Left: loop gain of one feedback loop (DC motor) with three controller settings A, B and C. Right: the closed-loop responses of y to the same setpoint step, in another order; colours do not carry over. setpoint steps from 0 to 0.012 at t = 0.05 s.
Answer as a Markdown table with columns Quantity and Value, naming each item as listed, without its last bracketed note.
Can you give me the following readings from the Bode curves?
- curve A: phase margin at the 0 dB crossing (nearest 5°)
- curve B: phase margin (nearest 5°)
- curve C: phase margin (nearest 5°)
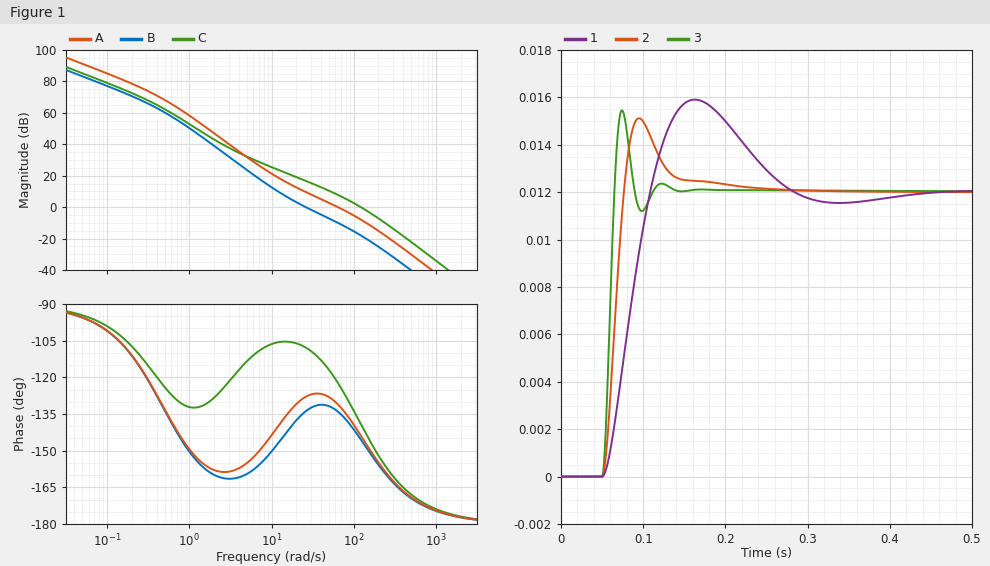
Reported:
| Quantity | Value |
|---|---|
| curve A: phase margin at the 0 dB crossing | 50° |
| curve B: phase margin | 45° |
| curve C: phase margin | 40° |
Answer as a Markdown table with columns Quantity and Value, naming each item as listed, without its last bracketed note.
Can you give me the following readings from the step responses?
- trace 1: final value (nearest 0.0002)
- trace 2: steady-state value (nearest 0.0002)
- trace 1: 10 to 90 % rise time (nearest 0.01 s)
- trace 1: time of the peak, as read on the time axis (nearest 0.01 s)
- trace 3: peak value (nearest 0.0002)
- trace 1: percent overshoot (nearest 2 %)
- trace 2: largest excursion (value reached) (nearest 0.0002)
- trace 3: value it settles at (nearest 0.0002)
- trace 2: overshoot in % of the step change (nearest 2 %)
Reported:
| Quantity | Value |
|---|---|
| trace 1: final value | 0.0120 |
| trace 2: steady-state value | 0.0120 |
| trace 1: 10 to 90 % rise time | 0.04 s |
| trace 1: time of the peak, as read on the time axis | 0.16 s |
| trace 3: peak value | 0.0154 |
| trace 1: percent overshoot | 32 % |
| trace 2: largest excursion (value reached) | 0.0152 |
| trace 3: value it settles at | 0.0120 |
| trace 2: overshoot in % of the step change | 26 % |
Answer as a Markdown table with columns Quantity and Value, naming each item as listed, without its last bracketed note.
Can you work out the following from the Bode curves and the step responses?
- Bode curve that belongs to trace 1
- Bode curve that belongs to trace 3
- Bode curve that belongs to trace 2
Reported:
| Quantity | Value |
|---|---|
| Bode curve that belongs to trace 1 | B |
| Bode curve that belongs to trace 3 | C |
| Bode curve that belongs to trace 2 | A |
